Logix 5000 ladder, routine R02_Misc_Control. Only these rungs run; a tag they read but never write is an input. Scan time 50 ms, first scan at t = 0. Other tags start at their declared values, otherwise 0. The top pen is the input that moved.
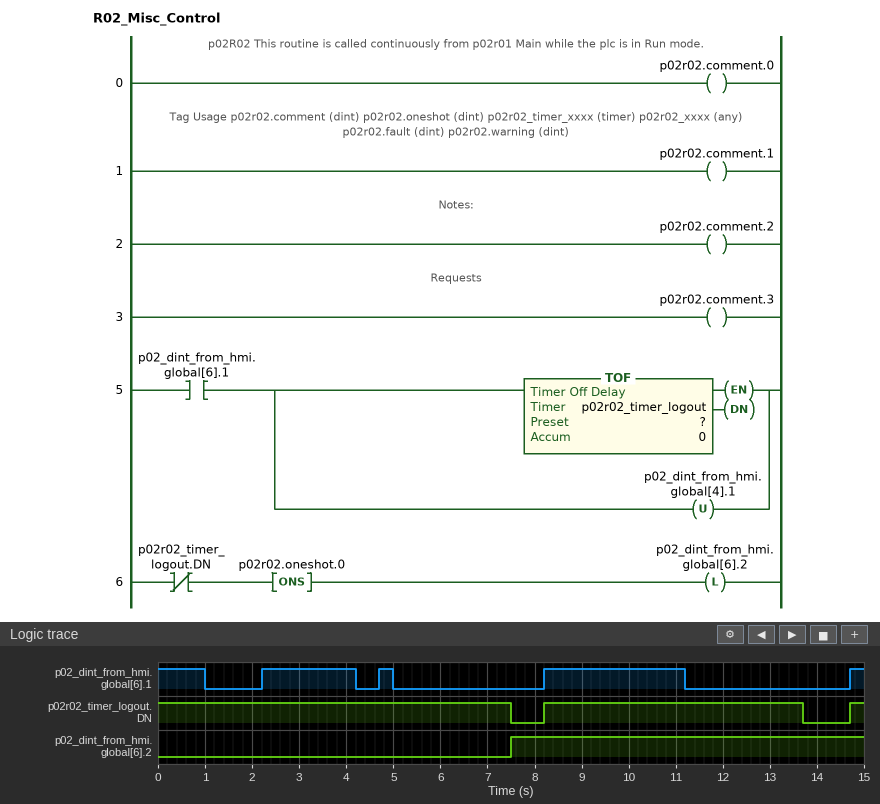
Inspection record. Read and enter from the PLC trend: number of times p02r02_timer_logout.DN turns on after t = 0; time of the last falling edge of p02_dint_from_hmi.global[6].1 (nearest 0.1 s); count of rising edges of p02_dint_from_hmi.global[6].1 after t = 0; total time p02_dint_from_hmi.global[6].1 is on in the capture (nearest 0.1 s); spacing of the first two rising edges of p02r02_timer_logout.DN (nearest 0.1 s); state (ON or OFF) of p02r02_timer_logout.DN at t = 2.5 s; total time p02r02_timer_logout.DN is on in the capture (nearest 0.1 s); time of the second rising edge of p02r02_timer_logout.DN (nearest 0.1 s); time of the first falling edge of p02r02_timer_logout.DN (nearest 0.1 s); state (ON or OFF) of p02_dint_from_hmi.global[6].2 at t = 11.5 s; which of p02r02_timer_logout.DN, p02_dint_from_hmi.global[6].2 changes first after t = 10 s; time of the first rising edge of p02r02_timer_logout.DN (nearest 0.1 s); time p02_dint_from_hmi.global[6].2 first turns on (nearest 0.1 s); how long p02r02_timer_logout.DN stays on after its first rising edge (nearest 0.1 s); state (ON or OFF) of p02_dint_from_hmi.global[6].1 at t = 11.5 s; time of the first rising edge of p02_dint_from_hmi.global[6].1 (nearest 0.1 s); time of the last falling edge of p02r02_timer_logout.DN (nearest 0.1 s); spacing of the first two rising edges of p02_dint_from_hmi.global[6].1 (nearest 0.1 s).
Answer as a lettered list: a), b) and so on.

a) 2
b) 11.2 s
c) 4
d) 6.6 s
e) 6.5 s
f) ON
g) 13.3 s
h) 14.7 s
i) 7.5 s
j) ON
k) p02r02_timer_logout.DN
l) 8.2 s
m) 7.5 s
n) 5.5 s
o) OFF
p) 2.2 s
q) 13.7 s
r) 2.5 s
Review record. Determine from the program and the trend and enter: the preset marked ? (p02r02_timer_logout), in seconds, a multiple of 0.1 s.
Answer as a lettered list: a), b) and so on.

a) 2.5 s
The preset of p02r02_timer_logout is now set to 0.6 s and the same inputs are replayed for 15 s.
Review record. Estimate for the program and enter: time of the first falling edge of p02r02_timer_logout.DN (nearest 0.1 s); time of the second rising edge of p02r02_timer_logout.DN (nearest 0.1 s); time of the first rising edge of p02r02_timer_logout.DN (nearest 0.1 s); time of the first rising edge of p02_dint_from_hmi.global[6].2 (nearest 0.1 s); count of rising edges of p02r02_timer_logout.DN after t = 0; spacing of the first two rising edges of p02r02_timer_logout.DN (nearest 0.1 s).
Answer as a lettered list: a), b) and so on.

a) 1.6 s
b) 8.2 s
c) 2.2 s
d) 1.6 s
e) 3
f) 6.0 s
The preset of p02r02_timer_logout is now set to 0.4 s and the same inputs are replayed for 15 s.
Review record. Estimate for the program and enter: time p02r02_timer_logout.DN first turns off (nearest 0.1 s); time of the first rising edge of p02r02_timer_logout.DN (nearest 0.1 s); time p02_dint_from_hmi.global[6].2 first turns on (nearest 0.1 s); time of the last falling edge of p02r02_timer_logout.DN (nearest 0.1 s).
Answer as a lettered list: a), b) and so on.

a) 1.4 s
b) 2.2 s
c) 1.4 s
d) 11.6 s
